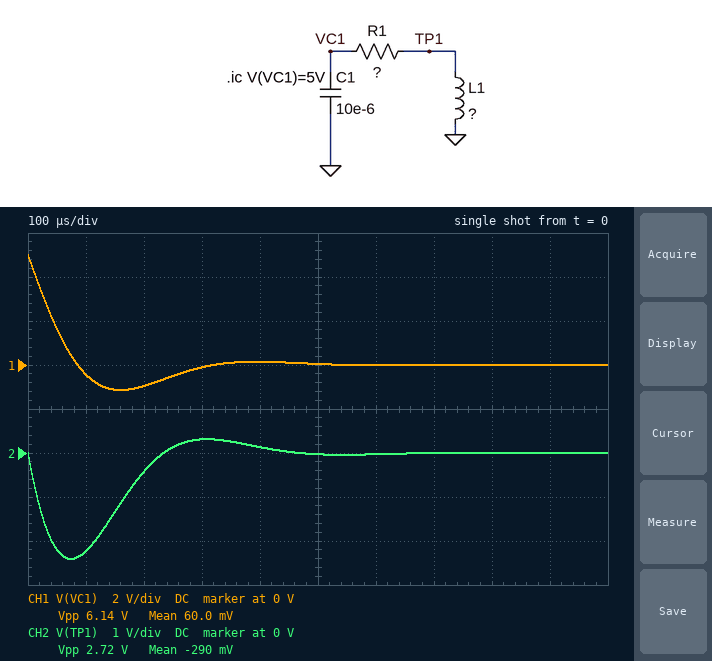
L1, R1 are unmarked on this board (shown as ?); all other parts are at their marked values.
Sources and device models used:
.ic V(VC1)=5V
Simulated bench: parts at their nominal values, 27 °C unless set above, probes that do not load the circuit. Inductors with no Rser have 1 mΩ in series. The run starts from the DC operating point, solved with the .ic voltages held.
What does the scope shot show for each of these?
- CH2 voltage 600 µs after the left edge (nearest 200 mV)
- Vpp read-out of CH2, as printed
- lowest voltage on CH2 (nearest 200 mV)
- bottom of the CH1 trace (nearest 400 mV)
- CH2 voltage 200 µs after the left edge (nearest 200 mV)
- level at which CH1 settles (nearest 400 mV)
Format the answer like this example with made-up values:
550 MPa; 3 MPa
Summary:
0 V; 2.72 V; -2.4 V; -1.2 V; -400 mV; 0 V
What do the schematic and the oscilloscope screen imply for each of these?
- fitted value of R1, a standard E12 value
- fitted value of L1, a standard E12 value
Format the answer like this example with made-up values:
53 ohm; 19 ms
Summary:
6.8 Ω; 390 µH
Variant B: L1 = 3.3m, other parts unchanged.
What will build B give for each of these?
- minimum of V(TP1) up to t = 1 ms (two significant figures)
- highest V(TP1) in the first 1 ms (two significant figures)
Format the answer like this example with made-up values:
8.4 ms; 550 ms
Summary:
-10 V; 5.6 V
